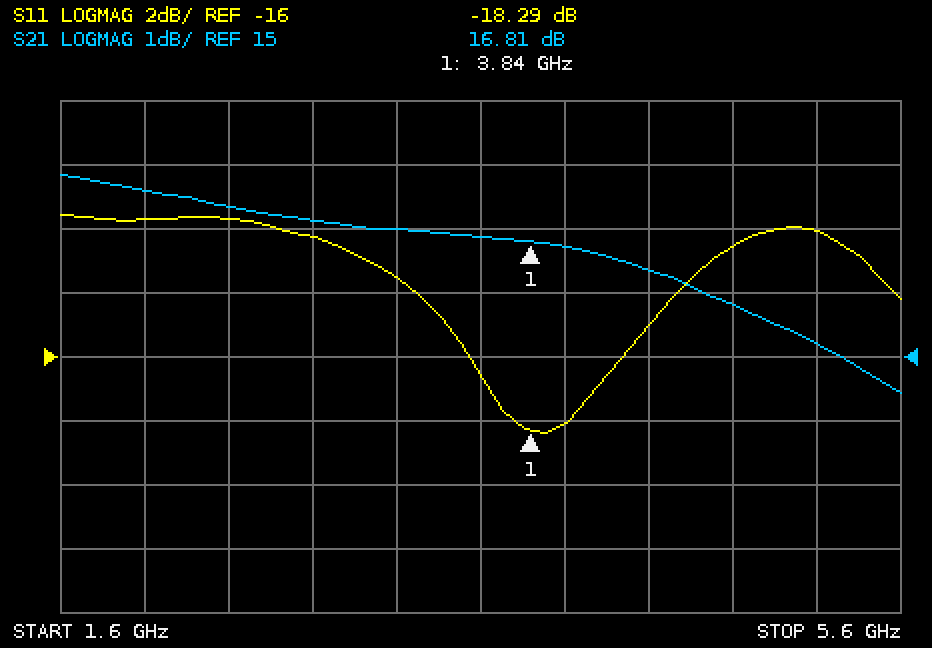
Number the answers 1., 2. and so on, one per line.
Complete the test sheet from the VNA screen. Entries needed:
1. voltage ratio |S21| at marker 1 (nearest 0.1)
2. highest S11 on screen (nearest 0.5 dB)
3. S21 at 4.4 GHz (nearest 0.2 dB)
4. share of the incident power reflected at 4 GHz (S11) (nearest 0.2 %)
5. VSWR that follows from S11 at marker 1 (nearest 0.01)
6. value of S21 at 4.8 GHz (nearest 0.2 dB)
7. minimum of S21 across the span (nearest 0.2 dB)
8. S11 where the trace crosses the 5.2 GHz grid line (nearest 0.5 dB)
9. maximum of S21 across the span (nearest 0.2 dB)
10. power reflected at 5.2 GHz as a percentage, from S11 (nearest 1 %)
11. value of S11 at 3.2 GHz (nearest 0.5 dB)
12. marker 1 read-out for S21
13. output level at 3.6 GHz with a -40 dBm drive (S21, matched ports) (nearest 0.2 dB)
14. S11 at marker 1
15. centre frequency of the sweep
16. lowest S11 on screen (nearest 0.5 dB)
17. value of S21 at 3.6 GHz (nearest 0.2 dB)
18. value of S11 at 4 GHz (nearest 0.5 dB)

1. 6.9
2. -11.5 dB
3. 16.4 dB
4. 1.6 %
5. 1.28
6. 15.8 dB
7. 14.4 dB
8. -12.0 dB
9. 17.8 dB
10. 6 %
11. -13.5 dB
12. 16.81 dB
13. -23.2 dBm
14. -18.29 dB
15. 3.6 GHz
16. -18.5 dB
17. 16.8 dB
18. -18.0 dB
